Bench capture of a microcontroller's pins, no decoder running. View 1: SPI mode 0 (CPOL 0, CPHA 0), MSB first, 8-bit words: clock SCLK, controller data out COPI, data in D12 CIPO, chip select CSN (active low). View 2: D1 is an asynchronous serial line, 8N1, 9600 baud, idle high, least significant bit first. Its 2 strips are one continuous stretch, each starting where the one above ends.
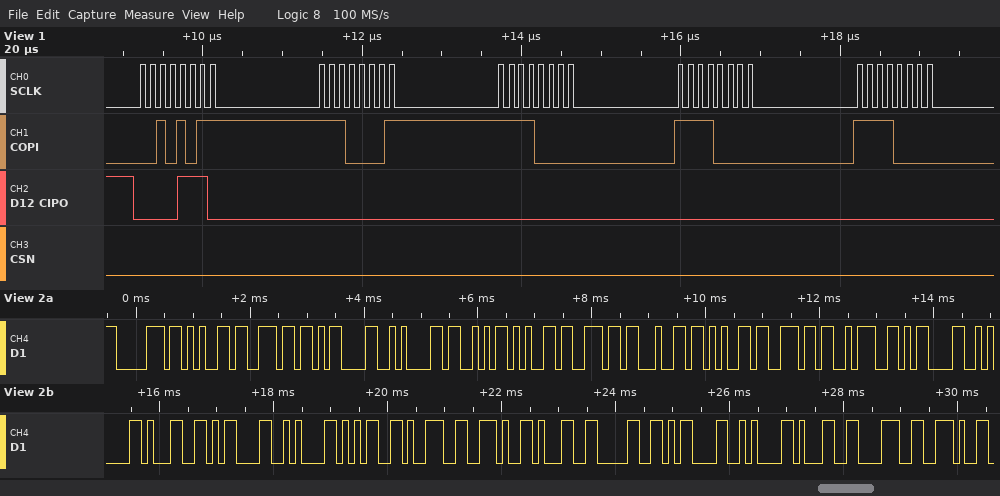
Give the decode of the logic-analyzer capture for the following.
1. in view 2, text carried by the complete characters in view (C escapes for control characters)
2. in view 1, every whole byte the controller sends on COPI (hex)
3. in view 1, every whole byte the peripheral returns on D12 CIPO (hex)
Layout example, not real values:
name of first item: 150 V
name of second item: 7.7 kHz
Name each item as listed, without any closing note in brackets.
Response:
in view 2, text carried by the complete characters in view: "pen\r\nSenden:\r\n1\r\n59.10\r\n18."
in view 1, every whole byte the controller sends on COPI: 0x2B 0xE1 0xF0 0xF0 0xF0
in view 1, every whole byte the peripheral returns on D12 CIPO: 0x0E 0x00 0x00 0x00 0x00
